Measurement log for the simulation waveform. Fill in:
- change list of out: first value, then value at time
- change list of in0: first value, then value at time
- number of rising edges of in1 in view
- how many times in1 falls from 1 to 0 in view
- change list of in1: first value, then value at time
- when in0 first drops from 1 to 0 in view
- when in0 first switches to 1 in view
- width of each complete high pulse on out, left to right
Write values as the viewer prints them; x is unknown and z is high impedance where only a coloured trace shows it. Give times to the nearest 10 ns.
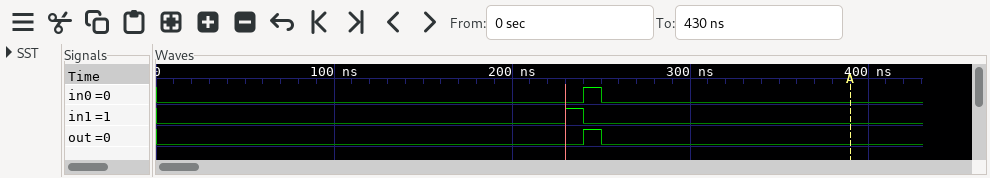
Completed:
0, 1 at 240 ns, 0 at 250 ns
0, 1 at 240 ns, 0 at 250 ns
1
1
0, 1 at 230 ns, 0 at 240 ns
250 ns
240 ns
10 ns
